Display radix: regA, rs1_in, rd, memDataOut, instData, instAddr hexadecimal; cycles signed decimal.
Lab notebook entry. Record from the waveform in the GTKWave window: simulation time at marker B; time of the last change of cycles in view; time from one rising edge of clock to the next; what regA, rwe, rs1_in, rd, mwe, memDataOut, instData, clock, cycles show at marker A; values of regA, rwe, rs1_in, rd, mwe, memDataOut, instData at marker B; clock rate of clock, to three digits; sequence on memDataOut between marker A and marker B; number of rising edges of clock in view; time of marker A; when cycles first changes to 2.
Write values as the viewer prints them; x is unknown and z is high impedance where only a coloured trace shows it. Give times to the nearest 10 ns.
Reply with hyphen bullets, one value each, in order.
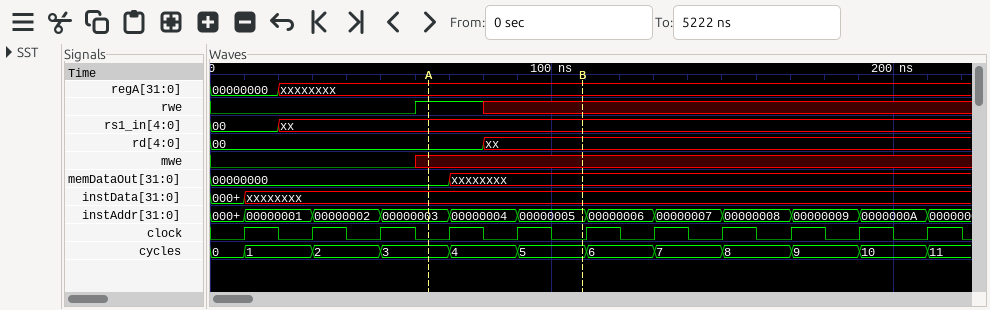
- 110 ns
- 210 ns
- 20 ns
- regA=xxxxxxxx, rwe=1, rs1_in=xx, rd=00, mwe=x, memDataOut=00000000, instData=xxxxxxxx, clock=0, cycles=3
- regA=xxxxxxxx, rwe=x, rs1_in=xx, rd=xx, mwe=x, memDataOut=xxxxxxxx, instData=xxxxxxxx
- 50.0 MHz
- 00000000, xxxxxxxx
- 11
- 60 ns
- 30 ns
